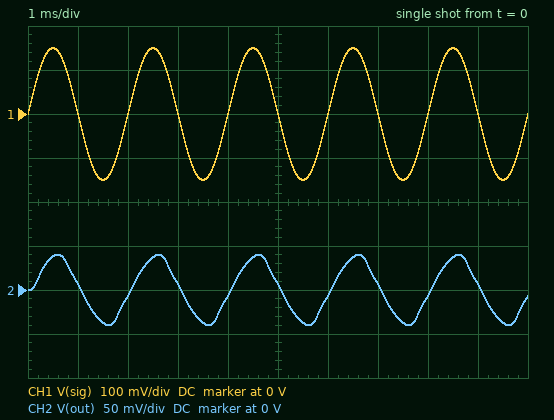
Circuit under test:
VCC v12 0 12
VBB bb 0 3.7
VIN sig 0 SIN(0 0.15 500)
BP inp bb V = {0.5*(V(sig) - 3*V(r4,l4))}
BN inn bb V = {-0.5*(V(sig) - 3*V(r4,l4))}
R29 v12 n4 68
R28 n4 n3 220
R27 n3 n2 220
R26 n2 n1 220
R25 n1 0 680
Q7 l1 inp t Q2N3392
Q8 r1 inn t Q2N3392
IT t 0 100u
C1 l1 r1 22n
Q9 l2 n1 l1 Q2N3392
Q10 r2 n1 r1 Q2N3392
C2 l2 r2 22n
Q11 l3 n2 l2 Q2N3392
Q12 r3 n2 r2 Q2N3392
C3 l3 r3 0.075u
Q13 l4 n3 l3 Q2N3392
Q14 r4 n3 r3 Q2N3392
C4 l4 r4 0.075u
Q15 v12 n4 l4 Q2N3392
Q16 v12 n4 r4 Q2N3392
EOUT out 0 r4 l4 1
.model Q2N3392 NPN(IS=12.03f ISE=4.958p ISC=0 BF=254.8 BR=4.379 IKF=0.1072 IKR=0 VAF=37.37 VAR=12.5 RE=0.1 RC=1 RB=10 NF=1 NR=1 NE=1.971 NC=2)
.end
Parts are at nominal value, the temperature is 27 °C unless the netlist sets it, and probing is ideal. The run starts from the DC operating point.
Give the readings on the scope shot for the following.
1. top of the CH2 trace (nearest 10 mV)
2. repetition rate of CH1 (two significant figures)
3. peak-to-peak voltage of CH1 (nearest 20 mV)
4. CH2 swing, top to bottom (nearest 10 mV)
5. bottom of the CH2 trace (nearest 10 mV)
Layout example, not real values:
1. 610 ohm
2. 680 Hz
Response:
1. 40 mV
2. 500 Hz
3. 300 mV
4. 80 mV
5. -40 mV
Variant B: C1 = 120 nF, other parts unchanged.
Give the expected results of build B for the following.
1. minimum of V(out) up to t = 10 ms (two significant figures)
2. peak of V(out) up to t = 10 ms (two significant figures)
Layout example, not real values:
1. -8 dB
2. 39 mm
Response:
1. -41 mV
2. 43 mV
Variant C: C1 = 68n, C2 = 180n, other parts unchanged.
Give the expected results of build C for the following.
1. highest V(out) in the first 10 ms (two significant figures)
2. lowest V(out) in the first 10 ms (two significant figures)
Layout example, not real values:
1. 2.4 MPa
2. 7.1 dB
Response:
1. 42 mV
2. -43 mV
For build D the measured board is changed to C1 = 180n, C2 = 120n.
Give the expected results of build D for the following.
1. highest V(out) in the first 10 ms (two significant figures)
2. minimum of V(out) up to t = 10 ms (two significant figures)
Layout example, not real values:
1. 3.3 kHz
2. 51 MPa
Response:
1. 43 mV
2. -43 mV
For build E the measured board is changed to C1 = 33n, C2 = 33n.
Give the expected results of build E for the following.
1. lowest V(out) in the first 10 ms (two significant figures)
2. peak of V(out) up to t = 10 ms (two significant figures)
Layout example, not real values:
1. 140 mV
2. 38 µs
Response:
1. -41 mV
2. 42 mV
